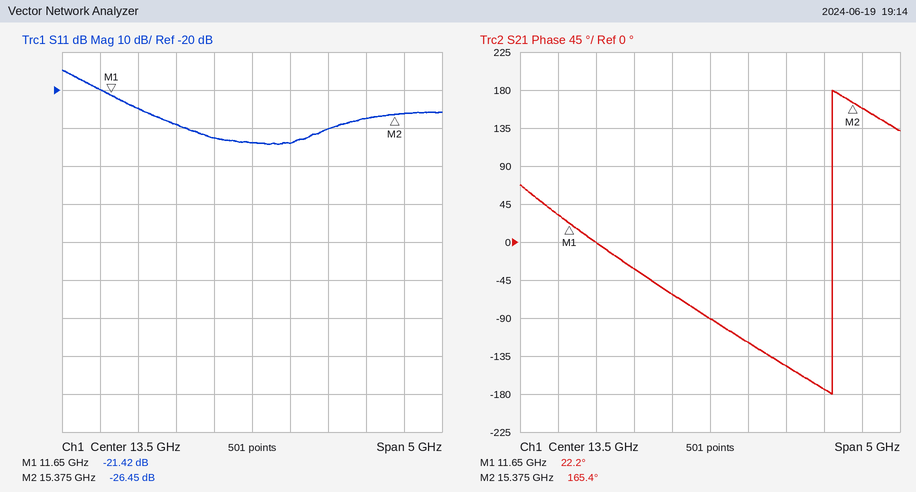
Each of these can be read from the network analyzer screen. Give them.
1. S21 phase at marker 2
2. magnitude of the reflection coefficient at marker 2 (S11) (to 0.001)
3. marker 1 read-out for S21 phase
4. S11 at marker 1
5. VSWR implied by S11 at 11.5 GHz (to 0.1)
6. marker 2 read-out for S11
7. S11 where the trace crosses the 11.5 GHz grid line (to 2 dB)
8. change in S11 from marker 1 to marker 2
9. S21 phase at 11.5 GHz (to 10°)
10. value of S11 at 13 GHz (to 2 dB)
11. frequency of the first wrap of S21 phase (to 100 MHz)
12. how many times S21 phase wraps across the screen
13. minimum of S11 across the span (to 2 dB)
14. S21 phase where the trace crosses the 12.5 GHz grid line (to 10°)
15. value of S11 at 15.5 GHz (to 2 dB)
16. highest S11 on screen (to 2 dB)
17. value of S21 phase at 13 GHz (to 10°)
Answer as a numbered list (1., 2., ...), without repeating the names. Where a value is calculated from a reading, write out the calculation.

1. 165.4°
2. 10^(-26.45/20) ≈ 0.048
3. 22.2°
4. -21.42 dB
5. |Γ| = 10^(-20/20) = 0.1000; VSWR = (1 + 0.1000)/(1 − 0.1000) ≈ 1.2
6. -26.45 dB
7. -20 dB
8. -26.45 − (-21.42) = -5.03 dB
9. 30°
10. -32 dB
11. 15.1 GHz
12. 1
13. -34 dB
14. -30°
15. -26 dB
16. -14 dB
17. -60°
